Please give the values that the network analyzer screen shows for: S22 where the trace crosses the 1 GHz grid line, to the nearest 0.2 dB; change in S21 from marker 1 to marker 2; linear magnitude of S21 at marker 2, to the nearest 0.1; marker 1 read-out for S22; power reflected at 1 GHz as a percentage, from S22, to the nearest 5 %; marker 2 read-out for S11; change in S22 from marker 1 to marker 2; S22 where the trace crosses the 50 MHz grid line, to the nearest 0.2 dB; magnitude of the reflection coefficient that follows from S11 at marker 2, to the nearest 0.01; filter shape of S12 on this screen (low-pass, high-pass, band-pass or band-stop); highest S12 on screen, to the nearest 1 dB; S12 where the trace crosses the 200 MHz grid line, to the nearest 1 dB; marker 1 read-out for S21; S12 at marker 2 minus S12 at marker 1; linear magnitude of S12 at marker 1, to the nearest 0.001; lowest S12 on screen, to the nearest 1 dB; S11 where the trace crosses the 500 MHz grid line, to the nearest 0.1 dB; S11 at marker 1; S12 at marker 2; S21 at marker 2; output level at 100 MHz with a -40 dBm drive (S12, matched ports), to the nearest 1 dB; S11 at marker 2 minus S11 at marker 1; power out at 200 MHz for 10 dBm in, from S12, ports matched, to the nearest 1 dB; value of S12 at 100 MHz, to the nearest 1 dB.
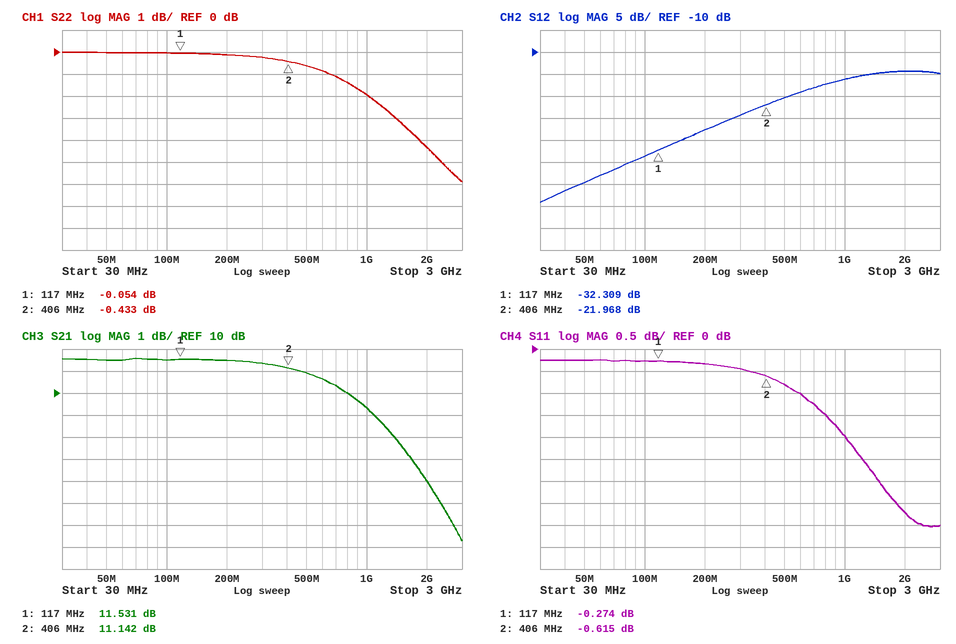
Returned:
-2.0 dB
-0.389 dB
3.6
-0.054 dB
65 %
-0.615 dB
-0.379 dB
0.0 dB
0.93
high-pass
-14 dB
-28 dB
11.531 dB
10.341 dB
0.024
-44 dB
-0.8 dB
-0.274 dB
-21.968 dB
11.142 dB
-74 dBm
-0.341 dB
-18 dBm
-34 dB
